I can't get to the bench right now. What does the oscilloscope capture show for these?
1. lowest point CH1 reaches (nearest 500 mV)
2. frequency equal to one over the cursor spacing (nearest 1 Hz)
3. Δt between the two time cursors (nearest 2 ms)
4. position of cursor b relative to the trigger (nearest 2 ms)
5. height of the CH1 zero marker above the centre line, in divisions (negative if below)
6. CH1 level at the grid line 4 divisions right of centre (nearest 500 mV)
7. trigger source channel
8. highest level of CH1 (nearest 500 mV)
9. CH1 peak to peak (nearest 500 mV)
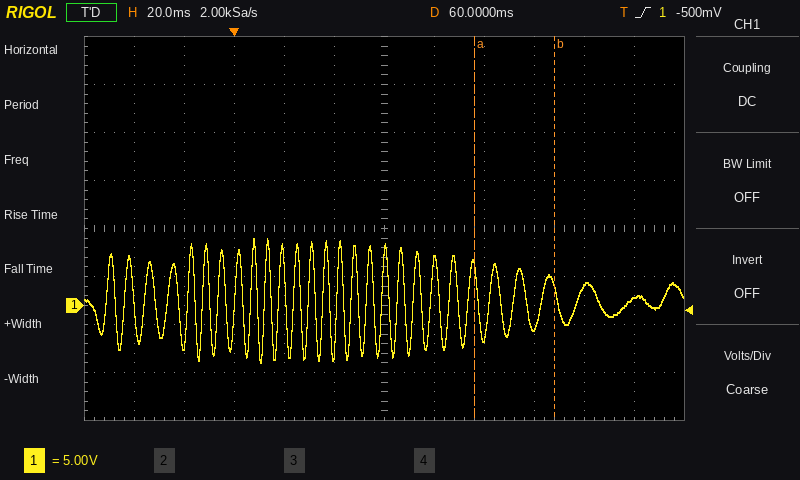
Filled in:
-6.0 V
31 Hz
32 ms
+128 ms
-1.6 div
2.0 V
CH1
7.0 V
13.0 V
